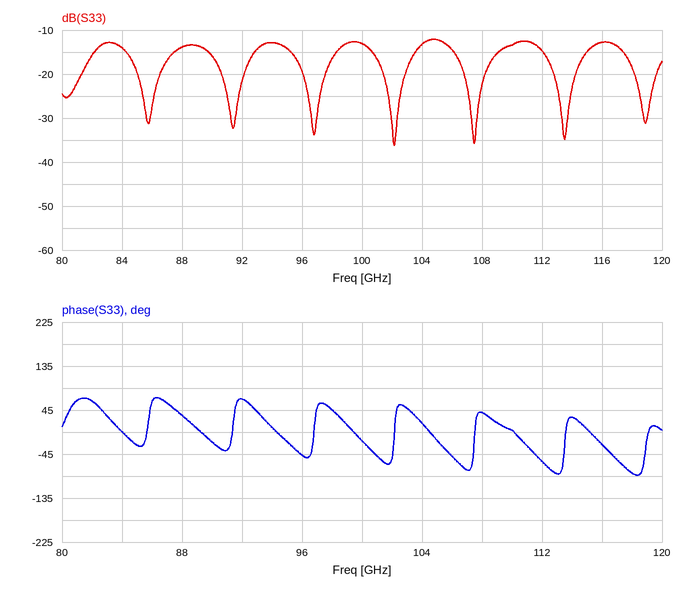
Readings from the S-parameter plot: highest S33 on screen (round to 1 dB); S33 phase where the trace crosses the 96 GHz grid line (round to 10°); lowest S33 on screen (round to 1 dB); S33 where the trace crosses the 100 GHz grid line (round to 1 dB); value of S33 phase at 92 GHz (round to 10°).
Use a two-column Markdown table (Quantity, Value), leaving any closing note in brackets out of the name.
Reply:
| Quantity | Value |
|---|---|
| highest S33 on screen | -12 dB |
| S33 phase where the trace crosses the 96 GHz grid line | -50° |
| lowest S33 on screen | -36 dB |
| S33 where the trace crosses the 100 GHz grid line | -13 dB |
| value of S33 phase at 92 GHz | 70° |
